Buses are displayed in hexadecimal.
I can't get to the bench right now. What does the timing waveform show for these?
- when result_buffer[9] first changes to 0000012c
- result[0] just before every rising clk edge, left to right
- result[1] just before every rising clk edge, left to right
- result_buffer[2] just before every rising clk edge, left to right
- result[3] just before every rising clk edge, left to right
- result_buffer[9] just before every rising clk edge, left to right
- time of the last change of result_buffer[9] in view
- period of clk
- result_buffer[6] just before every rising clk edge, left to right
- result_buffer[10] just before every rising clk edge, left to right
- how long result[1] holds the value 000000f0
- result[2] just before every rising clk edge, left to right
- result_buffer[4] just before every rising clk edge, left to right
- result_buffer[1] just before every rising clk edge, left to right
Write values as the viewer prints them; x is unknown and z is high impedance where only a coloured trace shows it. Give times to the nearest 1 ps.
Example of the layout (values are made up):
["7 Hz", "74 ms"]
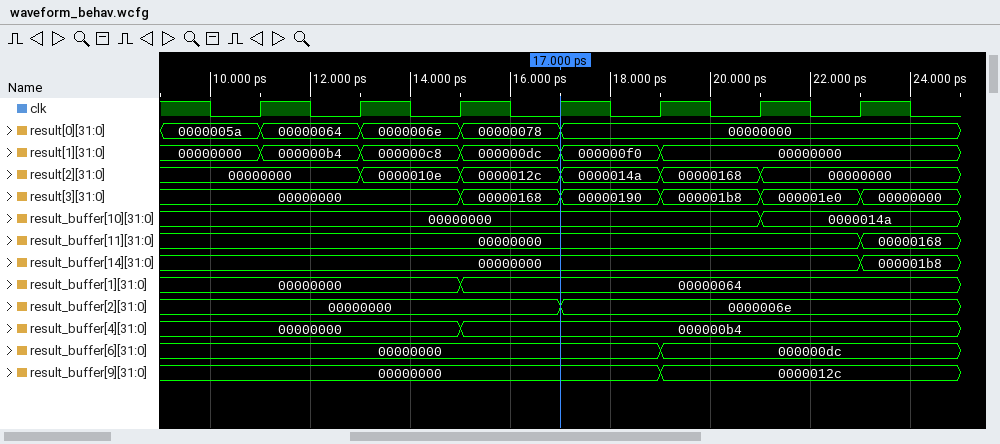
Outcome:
["19 ps", "0000005a, 00000064, 0000006e, 00000078, 00000000, 00000000, 00000000", "00000000, 000000b4, 000000c8, 000000dc, 000000f0, 00000000, 00000000", "00000000, 00000000, 00000000, 00000000, 0000006e, 0000006e, 0000006e", "00000000, 00000000, 00000000, 00000168, 00000190, 000001b8, 000001e0", "00000000, 00000000, 00000000, 00000000, 00000000, 0000012c, 0000012c", "19 ps", "2 ps", "00000000, 00000000, 00000000, 00000000, 00000000, 000000dc, 000000dc", "00000000, 00000000, 00000000, 00000000, 00000000, 00000000, 0000014a", "2 ps", "00000000, 00000000, 0000010e, 0000012c, 0000014a, 00000168, 00000000", "00000000, 00000000, 00000000, 000000b4, 000000b4, 000000b4, 000000b4", "00000000, 00000000, 00000000, 00000064, 00000064, 00000064, 00000064"]
